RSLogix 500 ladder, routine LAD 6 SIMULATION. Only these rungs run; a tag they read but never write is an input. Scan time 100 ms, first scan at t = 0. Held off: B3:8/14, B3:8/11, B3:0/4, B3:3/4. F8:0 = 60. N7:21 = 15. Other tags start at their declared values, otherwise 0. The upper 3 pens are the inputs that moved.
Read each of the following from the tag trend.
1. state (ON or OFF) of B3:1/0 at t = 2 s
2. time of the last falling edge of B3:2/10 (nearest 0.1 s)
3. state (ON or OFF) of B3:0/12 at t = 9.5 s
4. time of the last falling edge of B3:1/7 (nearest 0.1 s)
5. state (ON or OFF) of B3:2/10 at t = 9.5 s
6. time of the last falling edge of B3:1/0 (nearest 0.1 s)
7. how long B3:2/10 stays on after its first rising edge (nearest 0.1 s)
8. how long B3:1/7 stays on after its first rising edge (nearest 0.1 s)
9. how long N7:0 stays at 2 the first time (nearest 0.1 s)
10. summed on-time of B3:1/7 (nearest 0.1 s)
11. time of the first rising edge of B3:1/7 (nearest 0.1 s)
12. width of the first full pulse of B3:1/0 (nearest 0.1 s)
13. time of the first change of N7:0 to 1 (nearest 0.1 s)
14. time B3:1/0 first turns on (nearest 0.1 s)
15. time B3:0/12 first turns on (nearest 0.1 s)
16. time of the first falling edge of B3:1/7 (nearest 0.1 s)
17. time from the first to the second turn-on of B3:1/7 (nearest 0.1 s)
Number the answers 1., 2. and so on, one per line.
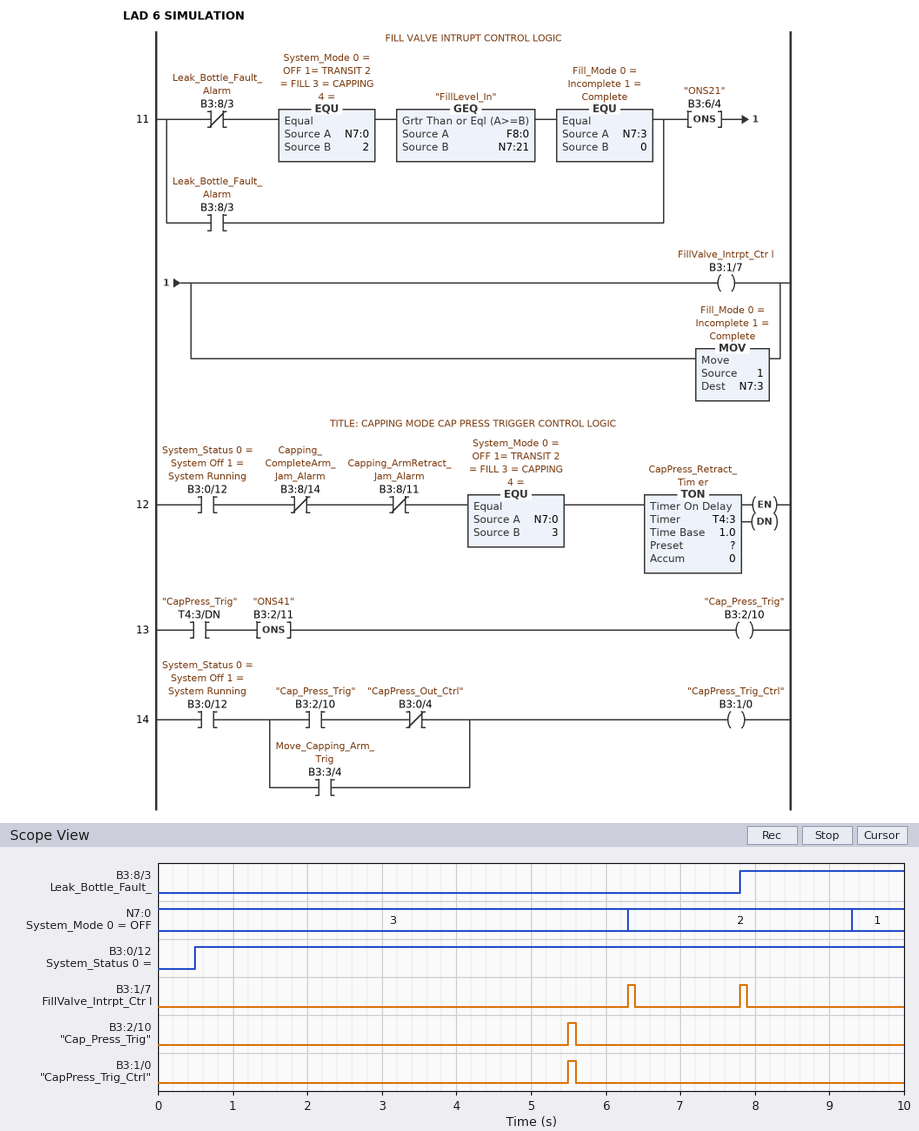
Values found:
1. OFF
2. 5.6 s
3. ON
4. 7.9 s
5. OFF
6. 5.6 s
7. 0.1 s
8. 0.1 s
9. 3.0 s
10. 0.2 s
11. 6.3 s
12. 0.1 s
13. 9.3 s
14. 5.5 s
15. 0.5 s
16. 6.4 s
17. 1.5 s
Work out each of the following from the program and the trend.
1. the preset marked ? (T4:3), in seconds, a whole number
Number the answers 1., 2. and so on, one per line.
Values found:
1. 5 s
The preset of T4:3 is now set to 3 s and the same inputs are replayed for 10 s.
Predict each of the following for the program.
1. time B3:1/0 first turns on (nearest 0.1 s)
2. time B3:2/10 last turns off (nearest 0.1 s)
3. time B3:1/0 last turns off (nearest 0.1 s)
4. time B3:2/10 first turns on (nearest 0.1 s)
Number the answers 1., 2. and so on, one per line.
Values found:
1. 3.5 s
2. 3.6 s
3. 3.6 s
4. 3.5 s
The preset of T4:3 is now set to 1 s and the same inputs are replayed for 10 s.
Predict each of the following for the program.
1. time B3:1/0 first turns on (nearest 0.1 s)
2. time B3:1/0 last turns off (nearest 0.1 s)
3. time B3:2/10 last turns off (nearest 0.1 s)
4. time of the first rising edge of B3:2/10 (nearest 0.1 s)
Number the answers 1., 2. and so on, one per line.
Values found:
1. 1.5 s
2. 1.6 s
3. 1.6 s
4. 1.5 s
